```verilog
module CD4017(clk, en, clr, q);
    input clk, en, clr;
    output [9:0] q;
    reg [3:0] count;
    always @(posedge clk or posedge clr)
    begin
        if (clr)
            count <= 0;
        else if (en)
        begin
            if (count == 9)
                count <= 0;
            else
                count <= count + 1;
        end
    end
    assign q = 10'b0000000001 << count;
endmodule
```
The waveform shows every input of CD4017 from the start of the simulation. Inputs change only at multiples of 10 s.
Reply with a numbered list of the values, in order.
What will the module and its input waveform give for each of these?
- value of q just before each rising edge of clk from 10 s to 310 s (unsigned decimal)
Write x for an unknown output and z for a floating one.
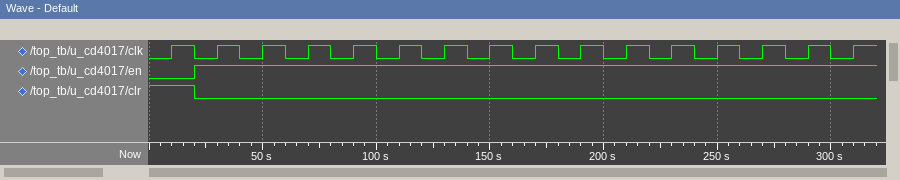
1. 1, 1, 2, 4, 8, 16, 32, 64, 128, 256, 512, 1, 2, 4, 8, 16
